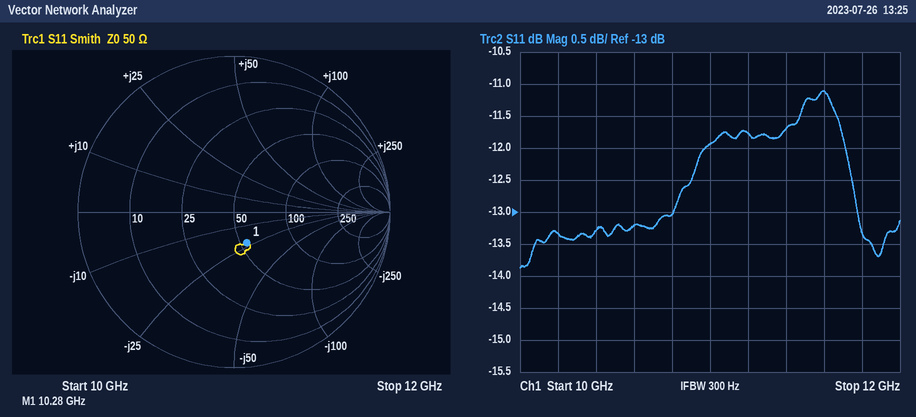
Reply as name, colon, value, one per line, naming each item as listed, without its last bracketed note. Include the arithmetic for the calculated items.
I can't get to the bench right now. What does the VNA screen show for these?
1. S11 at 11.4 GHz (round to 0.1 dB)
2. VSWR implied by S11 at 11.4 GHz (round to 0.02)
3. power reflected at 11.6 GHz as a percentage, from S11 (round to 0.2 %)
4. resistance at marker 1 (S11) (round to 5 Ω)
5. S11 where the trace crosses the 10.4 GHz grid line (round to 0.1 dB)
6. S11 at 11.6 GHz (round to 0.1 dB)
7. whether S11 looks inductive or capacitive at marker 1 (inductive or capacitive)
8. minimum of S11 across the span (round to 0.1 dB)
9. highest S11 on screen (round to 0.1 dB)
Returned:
S11 at 11.4 GHz: -11.7 dB
VSWR implied by S11 at 11.4 GHz: |Γ| = 10^(-11.7/20) = 0.2600; VSWR = (1 + 0.2600)/(1 − 0.2600) ≈ 1.70
power reflected at 11.6 GHz as a percentage, from S11: 10^(-11.1/10) ≈ 7.8 %
resistance at marker 1 (S11): 55 Ω
S11 where the trace crosses the 10.4 GHz grid line: -13.3 dB
S11 at 11.6 GHz: -11.1 dB
whether S11 looks inductive or capacitive at marker 1: capacitive
minimum of S11 across the span: -13.9 dB
highest S11 on screen: -11.1 dB
